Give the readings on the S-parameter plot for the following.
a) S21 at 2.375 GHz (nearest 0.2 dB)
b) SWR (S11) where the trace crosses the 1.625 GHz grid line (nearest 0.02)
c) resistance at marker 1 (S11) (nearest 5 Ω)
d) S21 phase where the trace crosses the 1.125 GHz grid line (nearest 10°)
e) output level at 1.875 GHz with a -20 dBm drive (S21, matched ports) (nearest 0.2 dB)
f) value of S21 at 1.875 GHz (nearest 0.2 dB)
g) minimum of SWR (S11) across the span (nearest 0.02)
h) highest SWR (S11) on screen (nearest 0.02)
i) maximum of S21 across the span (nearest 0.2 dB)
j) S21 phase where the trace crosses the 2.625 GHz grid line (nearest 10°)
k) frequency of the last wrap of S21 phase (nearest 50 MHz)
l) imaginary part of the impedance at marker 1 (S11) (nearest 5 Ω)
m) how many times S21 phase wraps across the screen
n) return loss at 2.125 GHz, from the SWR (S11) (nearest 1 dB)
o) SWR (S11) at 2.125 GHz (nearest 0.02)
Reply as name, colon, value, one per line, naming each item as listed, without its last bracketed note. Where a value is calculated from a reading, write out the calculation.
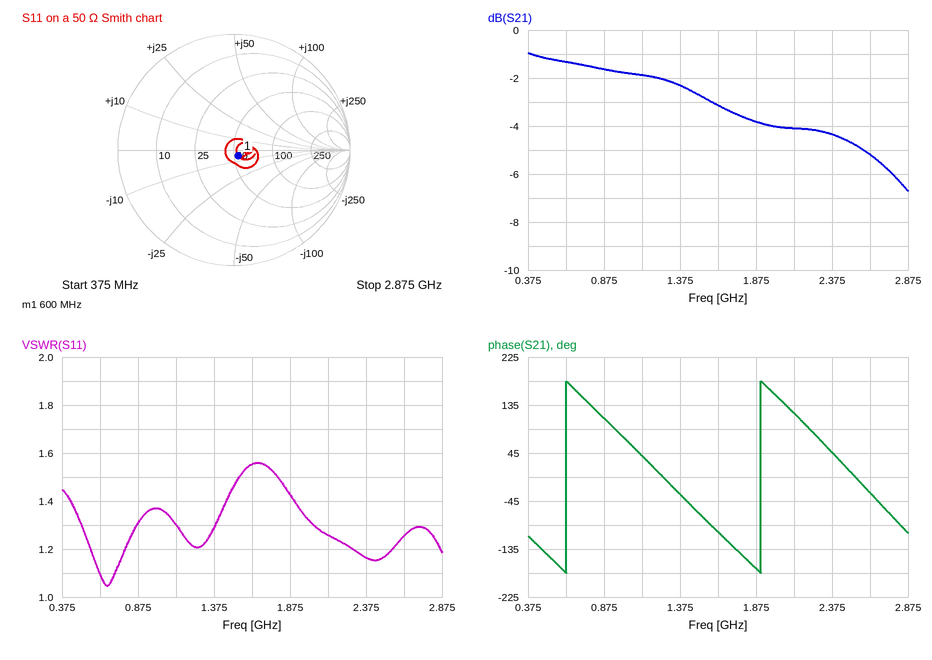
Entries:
S21 at 2.375 GHz: -4.4 dB
SWR (S11) where the trace crosses the 1.625 GHz grid line: 1.56
resistance at marker 1 (S11): 55 Ω
S21 phase where the trace crosses the 1.125 GHz grid line: 40°
output level at 1.875 GHz with a -20 dBm drive (S21, matched ports): -20 dBm + (-3.8 dB) = -23.8 dBm
value of S21 at 1.875 GHz: -3.8 dB
minimum of SWR (S11) across the span: 1.04
highest SWR (S11) on screen: 1.56
maximum of S21 across the span: -1.0 dB
S21 phase where the trace crosses the 2.625 GHz grid line: -30°
frequency of the last wrap of S21 phase: 1.90 GHz
imaginary part of the impedance at marker 1 (S11): -5 Ω
how many times S21 phase wraps across the screen: 2
return loss at 2.125 GHz, from the SWR (S11): −20 log10((1.26 − 1)/(1.26 + 1)) ≈ 19 dB
SWR (S11) at 2.125 GHz: 1.26
